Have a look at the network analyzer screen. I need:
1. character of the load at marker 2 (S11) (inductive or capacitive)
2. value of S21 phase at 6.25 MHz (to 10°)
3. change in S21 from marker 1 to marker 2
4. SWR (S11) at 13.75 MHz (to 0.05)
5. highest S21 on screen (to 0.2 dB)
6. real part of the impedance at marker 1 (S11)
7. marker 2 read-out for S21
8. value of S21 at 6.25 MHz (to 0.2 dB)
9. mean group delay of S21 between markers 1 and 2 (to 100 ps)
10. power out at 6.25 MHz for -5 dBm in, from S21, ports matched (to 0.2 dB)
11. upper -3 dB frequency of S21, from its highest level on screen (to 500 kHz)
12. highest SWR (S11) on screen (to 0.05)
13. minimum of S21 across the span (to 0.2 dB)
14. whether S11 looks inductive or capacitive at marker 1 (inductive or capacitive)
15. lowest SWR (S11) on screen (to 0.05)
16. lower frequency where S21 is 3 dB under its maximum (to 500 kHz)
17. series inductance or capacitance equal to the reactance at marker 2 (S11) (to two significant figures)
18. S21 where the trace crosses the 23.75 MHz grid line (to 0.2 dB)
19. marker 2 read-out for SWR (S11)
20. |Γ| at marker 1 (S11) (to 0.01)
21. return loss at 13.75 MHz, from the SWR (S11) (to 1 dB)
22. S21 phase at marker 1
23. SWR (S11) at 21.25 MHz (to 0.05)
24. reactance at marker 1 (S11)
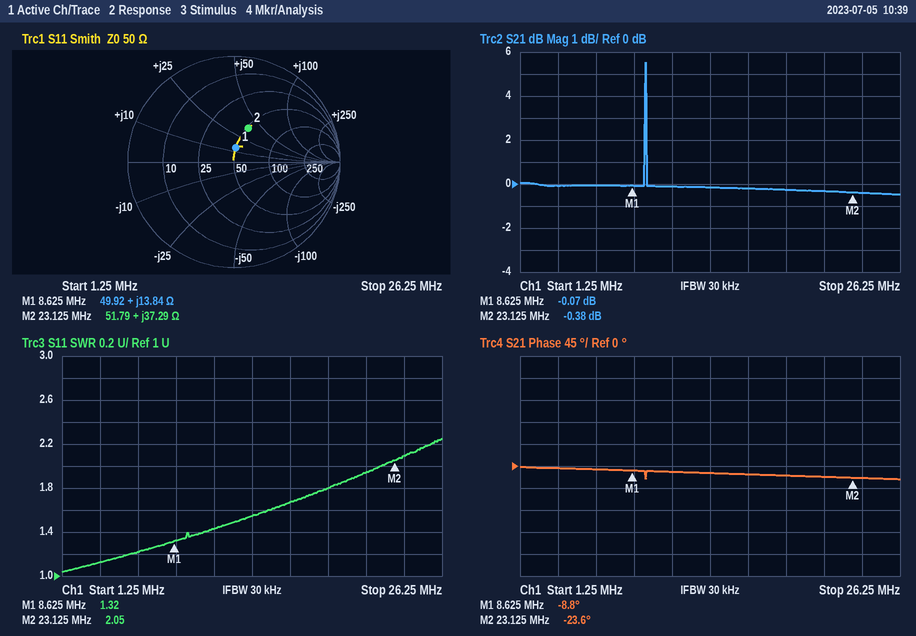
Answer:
inductive
-10°
-0.31 dB
1.55
5.6 dB
49.92 Ω
-0.38 dB
0.0 dB
2.8 ns
-5.0 dBm
9.5 MHz
2.25
-0.4 dB
inductive
1.05
9.5 MHz
260 nH
-0.4 dB
2.05
0.14
13 dB
-8.8°
1.95
+13.84 Ω
